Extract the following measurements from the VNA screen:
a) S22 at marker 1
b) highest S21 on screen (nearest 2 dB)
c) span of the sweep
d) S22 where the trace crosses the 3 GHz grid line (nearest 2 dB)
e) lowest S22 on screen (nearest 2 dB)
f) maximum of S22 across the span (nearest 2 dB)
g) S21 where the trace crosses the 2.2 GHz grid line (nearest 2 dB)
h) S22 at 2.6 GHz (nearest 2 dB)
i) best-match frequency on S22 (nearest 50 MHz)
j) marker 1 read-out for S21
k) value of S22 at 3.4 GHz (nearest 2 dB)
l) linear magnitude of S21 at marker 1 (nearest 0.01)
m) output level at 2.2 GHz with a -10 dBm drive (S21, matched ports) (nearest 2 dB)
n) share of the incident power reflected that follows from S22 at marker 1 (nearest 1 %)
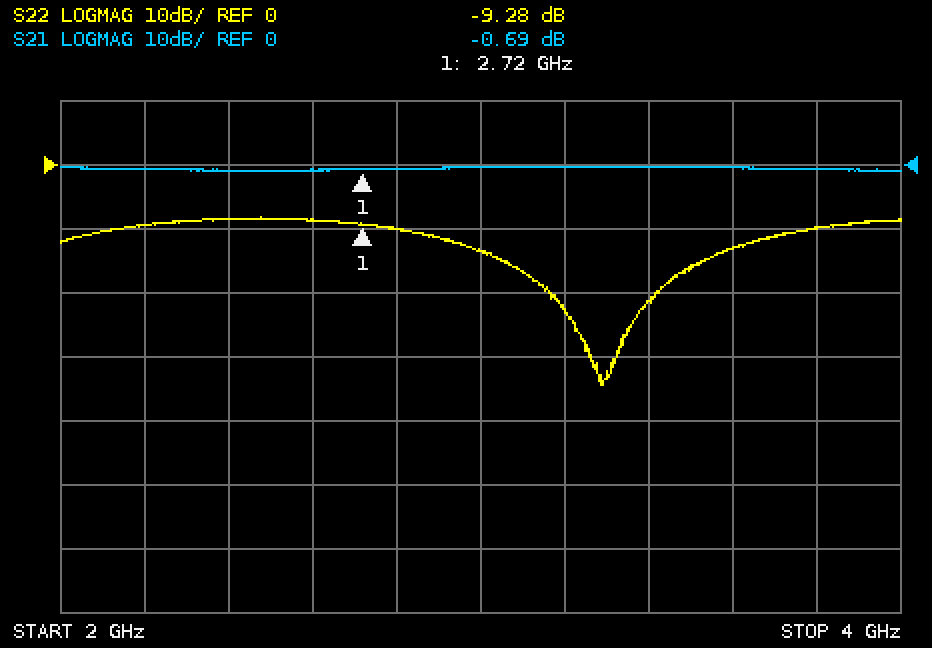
-9.28 dB
0 dB
2 GHz
-14 dB
-34 dB
-8 dB
0 dB
-8 dB
3.30 GHz
-0.69 dB
-22 dB
0.92
-10 dBm
12 %
